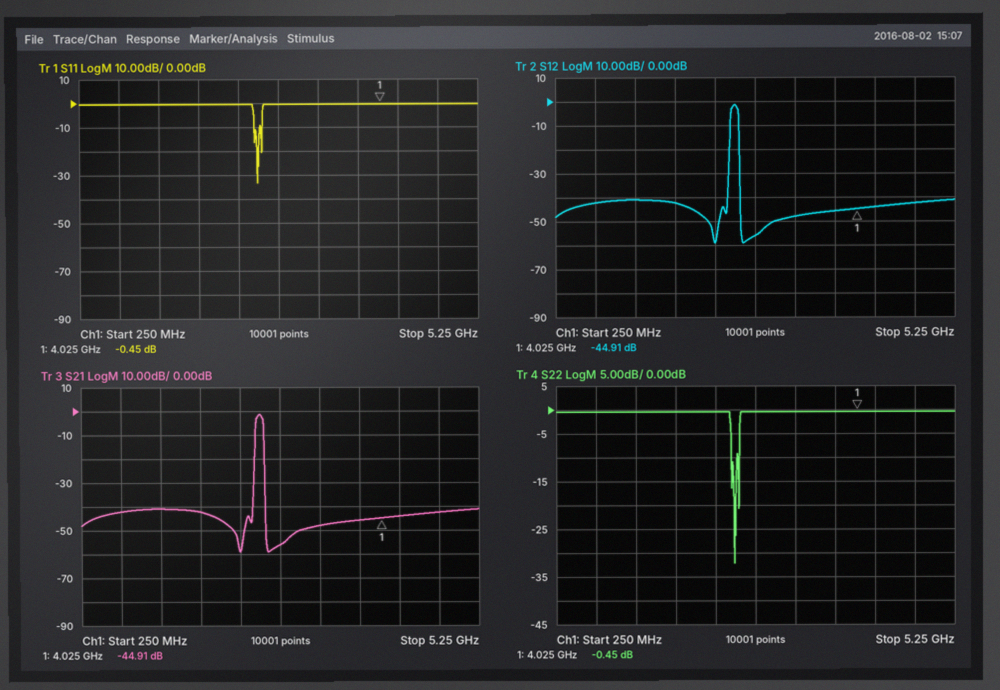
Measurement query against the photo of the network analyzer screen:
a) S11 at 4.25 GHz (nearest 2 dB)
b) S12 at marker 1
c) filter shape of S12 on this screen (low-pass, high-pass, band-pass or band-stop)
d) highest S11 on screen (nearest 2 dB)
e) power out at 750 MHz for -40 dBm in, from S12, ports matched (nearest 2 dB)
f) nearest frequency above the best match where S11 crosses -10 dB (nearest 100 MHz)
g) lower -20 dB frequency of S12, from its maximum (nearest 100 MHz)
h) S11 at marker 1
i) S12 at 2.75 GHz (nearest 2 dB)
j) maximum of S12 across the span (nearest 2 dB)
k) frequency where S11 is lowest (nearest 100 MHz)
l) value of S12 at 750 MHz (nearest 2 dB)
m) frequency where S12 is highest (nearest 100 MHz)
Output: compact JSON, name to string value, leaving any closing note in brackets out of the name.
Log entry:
{"S11 at 4.25 GHz": "0 dB", "S12 at marker 1": "-44.91 dB", "filter shape of S12 on this screen": "band-pass", "highest S11 on screen": "0 dB", "power out at 750 MHz for -40 dBm in, from S12, ports matched": "-82 dBm", "nearest frequency above the best match where S11 crosses -10 dB": "2.5 GHz", "lower -20 dB frequency of S12, from its maximum": "2.4 GHz", "S11 at marker 1": "-0.45 dB", "S12 at 2.75 GHz": "-56 dB", "maximum of S12 across the span": "-2 dB", "frequency where S11 is lowest": "2.5 GHz", "value of S12 at 750 MHz": "-42 dB", "frequency where S12 is highest": "2.5 GHz"}
